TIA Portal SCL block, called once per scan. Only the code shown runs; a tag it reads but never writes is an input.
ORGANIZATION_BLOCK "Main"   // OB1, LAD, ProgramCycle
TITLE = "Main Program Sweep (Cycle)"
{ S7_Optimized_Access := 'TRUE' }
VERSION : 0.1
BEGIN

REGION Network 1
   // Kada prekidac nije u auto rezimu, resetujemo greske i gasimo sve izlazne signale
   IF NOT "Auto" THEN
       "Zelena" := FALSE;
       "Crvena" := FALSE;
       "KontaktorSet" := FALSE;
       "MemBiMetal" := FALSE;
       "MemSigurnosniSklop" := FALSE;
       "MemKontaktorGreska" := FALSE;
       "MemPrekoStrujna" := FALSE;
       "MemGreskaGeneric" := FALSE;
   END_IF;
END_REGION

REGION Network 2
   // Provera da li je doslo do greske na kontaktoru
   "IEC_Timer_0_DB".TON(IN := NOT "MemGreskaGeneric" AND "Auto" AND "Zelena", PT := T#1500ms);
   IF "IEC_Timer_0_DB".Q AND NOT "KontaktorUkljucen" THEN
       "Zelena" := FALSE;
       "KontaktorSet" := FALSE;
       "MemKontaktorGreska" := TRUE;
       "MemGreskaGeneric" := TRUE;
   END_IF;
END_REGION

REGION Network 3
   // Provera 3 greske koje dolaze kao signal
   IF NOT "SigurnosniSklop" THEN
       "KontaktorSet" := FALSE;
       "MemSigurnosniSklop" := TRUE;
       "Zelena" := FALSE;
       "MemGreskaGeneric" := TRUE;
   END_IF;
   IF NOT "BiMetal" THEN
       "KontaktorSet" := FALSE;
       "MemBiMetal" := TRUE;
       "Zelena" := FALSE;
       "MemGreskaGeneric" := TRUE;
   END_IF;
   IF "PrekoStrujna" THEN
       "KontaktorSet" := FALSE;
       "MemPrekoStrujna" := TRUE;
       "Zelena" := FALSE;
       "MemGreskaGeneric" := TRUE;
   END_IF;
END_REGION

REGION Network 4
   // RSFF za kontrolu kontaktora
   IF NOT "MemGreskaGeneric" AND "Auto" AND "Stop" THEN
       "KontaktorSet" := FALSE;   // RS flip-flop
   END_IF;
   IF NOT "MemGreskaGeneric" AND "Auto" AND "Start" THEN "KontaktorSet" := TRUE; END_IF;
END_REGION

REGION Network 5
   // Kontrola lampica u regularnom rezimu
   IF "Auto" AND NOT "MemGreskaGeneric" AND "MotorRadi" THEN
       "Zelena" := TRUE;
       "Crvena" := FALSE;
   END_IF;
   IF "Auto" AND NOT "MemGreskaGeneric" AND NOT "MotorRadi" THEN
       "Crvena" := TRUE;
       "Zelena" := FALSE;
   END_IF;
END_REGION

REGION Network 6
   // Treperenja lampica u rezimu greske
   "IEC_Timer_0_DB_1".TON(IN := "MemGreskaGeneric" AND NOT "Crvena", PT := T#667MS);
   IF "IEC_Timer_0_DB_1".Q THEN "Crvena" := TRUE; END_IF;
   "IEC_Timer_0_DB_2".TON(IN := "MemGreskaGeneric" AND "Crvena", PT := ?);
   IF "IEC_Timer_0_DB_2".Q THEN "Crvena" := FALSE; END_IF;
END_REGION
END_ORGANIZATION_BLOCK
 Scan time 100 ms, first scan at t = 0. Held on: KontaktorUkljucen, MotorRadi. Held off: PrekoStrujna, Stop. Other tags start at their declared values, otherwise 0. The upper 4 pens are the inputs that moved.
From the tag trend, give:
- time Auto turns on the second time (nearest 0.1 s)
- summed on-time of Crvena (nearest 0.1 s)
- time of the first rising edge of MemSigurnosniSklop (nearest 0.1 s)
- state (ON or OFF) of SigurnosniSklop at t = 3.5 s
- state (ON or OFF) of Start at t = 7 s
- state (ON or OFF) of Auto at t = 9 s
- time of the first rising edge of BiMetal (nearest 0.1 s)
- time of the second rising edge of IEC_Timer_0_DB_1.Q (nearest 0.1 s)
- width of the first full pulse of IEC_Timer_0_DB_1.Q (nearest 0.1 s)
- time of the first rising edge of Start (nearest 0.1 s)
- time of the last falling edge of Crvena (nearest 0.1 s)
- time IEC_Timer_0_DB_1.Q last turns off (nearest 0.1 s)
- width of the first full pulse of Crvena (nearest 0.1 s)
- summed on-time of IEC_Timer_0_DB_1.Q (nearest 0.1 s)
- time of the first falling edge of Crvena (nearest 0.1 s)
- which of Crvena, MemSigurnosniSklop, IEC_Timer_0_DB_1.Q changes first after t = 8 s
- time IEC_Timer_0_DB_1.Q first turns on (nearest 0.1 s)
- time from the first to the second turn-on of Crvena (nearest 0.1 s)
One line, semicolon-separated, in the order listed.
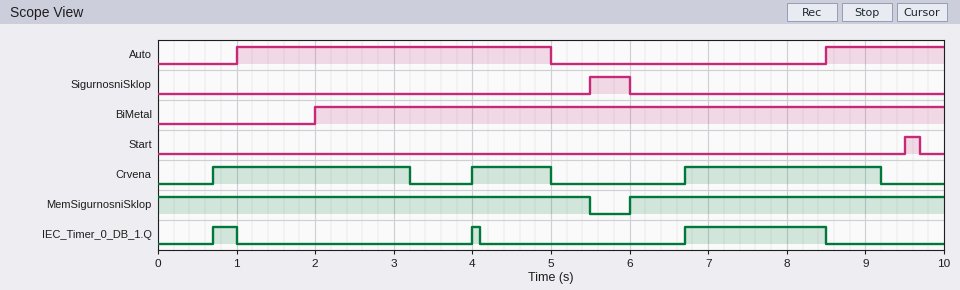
8.5 s; 6.0 s; 6.0 s; OFF; OFF; ON; 2.0 s; 4.0 s; 0.3 s; 9.5 s; 9.2 s; 8.5 s; 2.5 s; 2.2 s; 3.2 s; IEC_Timer_0_DB_1.Q; 0.7 s; 3.3 s
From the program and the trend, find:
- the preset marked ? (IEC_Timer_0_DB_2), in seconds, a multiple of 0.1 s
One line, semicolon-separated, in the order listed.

2.5 s
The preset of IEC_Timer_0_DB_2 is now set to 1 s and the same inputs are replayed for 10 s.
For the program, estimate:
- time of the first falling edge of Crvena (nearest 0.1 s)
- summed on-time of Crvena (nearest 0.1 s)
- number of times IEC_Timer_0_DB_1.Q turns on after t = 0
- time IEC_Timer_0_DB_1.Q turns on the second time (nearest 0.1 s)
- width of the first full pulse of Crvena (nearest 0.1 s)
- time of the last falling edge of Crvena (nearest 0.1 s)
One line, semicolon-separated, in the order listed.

1.7 s; 3.7 s; 4; 2.5 s; 1.0 s; 7.7 s
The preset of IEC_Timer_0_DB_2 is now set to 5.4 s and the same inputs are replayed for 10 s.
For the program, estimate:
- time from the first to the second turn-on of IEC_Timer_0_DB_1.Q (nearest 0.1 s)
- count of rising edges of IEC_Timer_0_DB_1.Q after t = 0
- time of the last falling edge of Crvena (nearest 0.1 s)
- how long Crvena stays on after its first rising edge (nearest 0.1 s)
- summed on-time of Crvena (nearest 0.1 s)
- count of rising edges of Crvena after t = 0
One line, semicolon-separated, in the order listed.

6.0 s; 2; 5.0 s; 4.3 s; 7.6 s; 2
